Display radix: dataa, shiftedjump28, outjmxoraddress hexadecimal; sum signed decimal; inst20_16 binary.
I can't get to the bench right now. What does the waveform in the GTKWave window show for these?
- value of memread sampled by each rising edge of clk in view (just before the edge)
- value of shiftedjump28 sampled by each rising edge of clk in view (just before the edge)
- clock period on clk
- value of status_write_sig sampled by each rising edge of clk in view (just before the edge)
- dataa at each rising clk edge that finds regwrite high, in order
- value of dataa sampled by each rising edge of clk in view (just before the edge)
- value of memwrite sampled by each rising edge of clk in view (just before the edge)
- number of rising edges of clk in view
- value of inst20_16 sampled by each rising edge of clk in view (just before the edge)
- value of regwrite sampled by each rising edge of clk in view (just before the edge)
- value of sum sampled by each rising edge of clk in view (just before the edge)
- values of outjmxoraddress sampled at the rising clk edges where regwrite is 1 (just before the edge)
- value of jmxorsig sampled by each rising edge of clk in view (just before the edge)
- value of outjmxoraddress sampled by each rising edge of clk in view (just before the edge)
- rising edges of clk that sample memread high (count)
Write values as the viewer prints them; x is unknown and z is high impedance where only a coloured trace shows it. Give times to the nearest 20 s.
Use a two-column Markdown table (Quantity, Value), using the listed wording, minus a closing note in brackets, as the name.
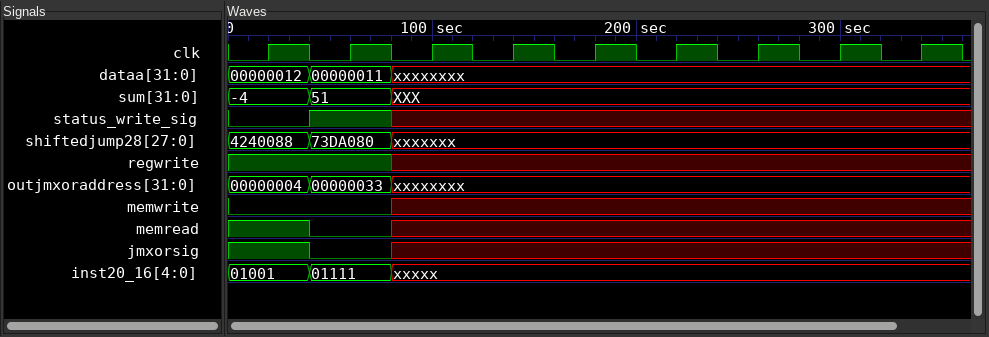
| Quantity | Value |
|---|---|
| value of memread sampled by each rising edge of clk in view | 1 0 x x x x x x x |
| value of shiftedjump28 sampled by each rising edge of clk in view | 4240088, 73DA080, xxxxxxx, xxxxxxx, xxxxxxx, xxxxxxx, xxxxxxx, xxxxxxx, xxxxxxx |
| clock period on clk | 40 s |
| value of status_write_sig sampled by each rising edge of clk in view | 0 1 x x x x x x x |
| dataa at each rising clk edge that finds regwrite high, in order | 00000012, 00000011 |
| value of dataa sampled by each rising edge of clk in view | 00000012, 00000011, xxxxxxxx, xxxxxxxx, xxxxxxxx, xxxxxxxx, xxxxxxxx, xxxxxxxx, xxxxxxxx |
| value of memwrite sampled by each rising edge of clk in view | 0 0 x x x x x x x |
| number of rising edges of clk in view | 9 |
| value of inst20_16 sampled by each rising edge of clk in view | 01001, 01111, xxxxx, xxxxx, xxxxx, xxxxx, xxxxx, xxxxx, xxxxx |
| value of regwrite sampled by each rising edge of clk in view | 1 1 x x x x x x x |
| value of sum sampled by each rising edge of clk in view | -4, 51, XXX, XXX, XXX, XXX, XXX, XXX, XXX |
| values of outjmxoraddress sampled at the rising clk edges where regwrite is 1 | 00000004, 00000033 |
| value of jmxorsig sampled by each rising edge of clk in view | 1 0 x x x x x x x |
| value of outjmxoraddress sampled by each rising edge of clk in view | 00000004, 00000033, xxxxxxxx, xxxxxxxx, xxxxxxxx, xxxxxxxx, xxxxxxxx, xxxxxxxx, xxxxxxxx |
| rising edges of clk that sample memread high | 1 |
